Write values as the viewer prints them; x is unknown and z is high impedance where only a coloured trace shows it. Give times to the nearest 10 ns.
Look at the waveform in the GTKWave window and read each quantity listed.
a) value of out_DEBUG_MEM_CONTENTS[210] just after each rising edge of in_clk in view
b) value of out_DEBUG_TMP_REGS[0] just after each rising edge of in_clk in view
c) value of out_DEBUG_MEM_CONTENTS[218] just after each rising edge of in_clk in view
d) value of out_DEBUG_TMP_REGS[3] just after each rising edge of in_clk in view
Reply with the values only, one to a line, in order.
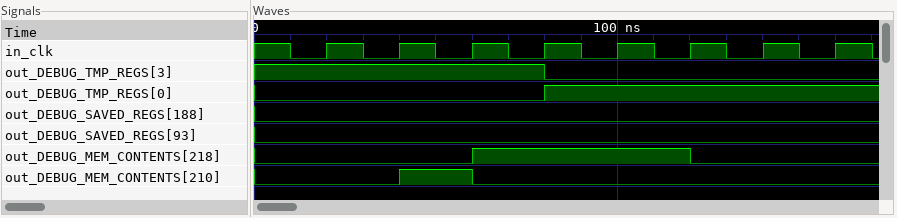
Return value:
0 1 0 0 0 0 0 0
0 0 0 1 1 1 1 1
0 0 1 1 1 0 0 0
1 1 1 0 0 0 0 0
